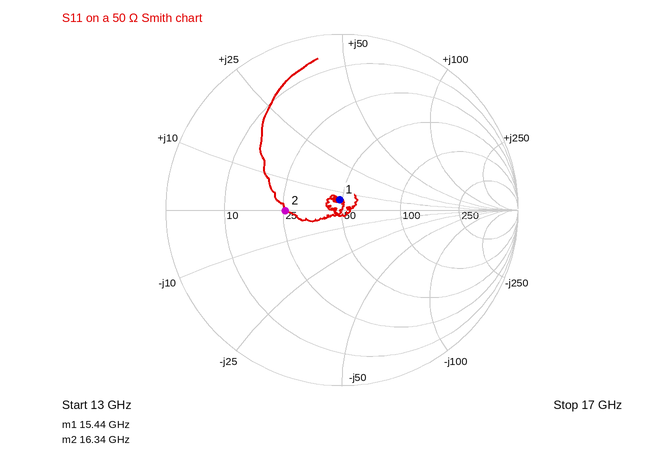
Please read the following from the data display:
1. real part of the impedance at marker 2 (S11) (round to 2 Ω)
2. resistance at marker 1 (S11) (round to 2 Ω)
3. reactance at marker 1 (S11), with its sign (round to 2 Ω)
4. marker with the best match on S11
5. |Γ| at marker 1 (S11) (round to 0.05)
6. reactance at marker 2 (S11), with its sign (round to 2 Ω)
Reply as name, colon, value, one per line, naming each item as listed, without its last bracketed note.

real part of the impedance at marker 2 (S11): 26 Ω
resistance at marker 1 (S11): 48 Ω
reactance at marker 1 (S11), with its sign: +6 Ω
marker with the best match on S11: marker 1
|Γ| at marker 1 (S11): 0.05
reactance at marker 2 (S11), with its sign: 0 Ω
